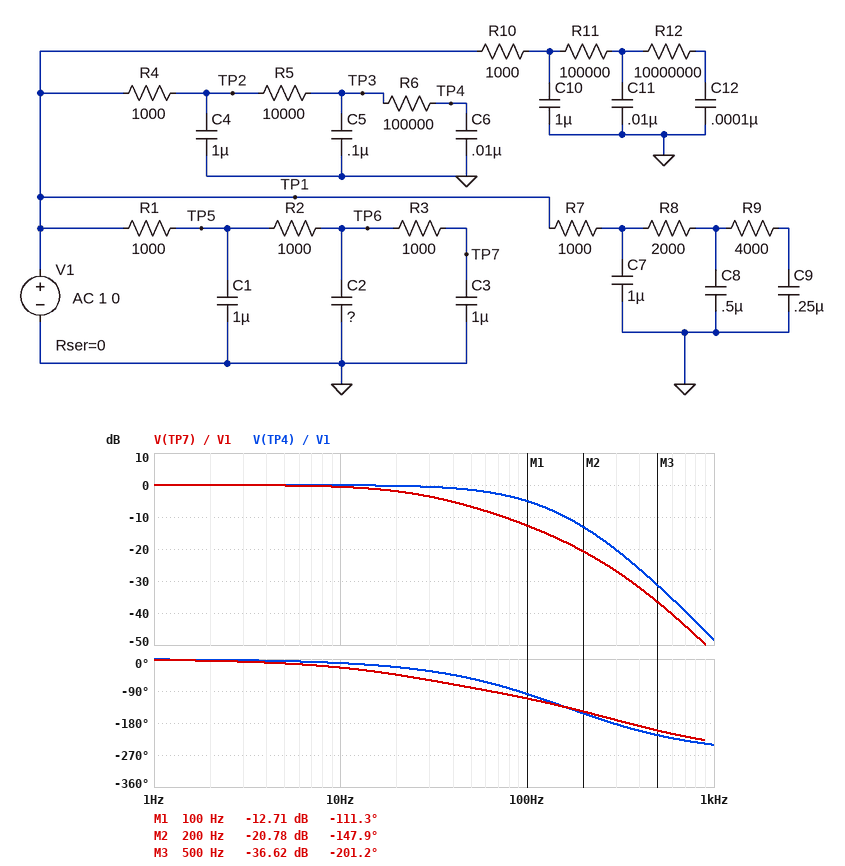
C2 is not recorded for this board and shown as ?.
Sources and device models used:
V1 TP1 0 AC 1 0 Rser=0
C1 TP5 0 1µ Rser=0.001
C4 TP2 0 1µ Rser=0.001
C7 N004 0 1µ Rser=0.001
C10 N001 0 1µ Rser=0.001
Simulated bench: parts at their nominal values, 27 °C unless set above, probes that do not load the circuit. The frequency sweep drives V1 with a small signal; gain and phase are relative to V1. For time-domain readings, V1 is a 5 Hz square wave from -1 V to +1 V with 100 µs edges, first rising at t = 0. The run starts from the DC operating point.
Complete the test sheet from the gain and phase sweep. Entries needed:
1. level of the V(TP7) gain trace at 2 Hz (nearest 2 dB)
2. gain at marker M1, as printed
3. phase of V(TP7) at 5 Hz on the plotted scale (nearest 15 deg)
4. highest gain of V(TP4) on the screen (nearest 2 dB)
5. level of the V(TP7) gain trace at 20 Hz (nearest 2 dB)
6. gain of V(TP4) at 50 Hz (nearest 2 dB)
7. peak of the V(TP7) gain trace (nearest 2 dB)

0 dB
-12.71 dB
-15 deg
0 dB
-2 dB
-2 dB
0 dB
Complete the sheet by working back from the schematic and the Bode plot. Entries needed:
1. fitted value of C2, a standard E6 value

1.5 µF
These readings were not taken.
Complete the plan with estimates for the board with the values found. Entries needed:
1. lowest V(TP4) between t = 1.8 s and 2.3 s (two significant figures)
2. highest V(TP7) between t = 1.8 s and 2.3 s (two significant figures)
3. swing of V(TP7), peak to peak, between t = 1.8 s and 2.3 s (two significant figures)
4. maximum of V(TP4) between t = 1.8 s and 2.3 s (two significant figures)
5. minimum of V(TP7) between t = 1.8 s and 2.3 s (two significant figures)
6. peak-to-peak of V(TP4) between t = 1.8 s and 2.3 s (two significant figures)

-1.0 V
1.0 V
2.0 V
1.0 V
-1.0 V
2.0 V
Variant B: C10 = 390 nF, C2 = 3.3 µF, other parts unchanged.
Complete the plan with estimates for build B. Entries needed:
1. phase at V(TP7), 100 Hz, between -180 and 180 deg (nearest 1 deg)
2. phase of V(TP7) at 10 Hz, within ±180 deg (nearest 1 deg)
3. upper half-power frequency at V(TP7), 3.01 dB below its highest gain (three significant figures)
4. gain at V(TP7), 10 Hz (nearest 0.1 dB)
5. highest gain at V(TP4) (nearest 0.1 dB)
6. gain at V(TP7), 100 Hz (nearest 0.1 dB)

-122 deg
-35 deg
16.8 Hz
-1.3 dB
0 dB
-16.8 dB
